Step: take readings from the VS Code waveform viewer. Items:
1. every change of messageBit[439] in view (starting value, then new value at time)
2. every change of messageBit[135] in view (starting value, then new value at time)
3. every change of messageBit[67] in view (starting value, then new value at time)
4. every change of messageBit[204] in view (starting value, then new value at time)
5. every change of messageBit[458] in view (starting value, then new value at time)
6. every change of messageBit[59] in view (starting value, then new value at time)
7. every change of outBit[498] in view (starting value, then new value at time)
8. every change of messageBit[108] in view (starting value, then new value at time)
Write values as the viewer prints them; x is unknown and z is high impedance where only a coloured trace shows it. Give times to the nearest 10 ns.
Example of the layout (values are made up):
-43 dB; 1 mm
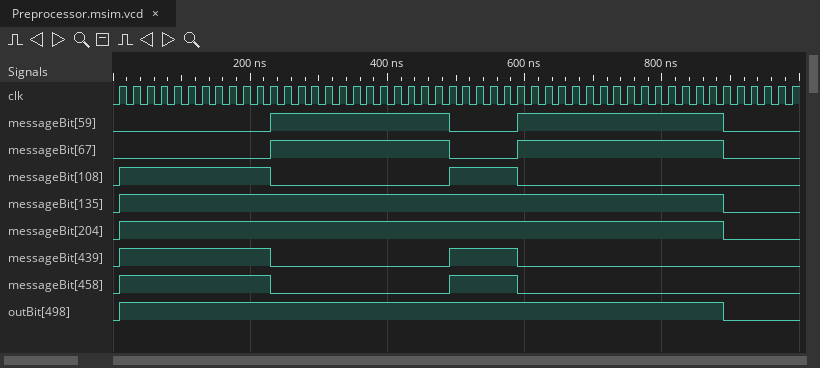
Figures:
0, 1 at 10 ns, 0 at 230 ns, 1 at 490 ns, 0 at 590 ns; 0, 1 at 10 ns, 0 at 890 ns; 0, 1 at 230 ns, 0 at 490 ns, 1 at 590 ns, 0 at 890 ns; 0, 1 at 10 ns, 0 at 890 ns; 0, 1 at 10 ns, 0 at 230 ns, 1 at 490 ns, 0 at 590 ns; 0, 1 at 230 ns, 0 at 490 ns, 1 at 590 ns, 0 at 890 ns; 0, 1 at 10 ns, 0 at 890 ns; 0, 1 at 10 ns, 0 at 230 ns, 1 at 490 ns, 0 at 590 ns
